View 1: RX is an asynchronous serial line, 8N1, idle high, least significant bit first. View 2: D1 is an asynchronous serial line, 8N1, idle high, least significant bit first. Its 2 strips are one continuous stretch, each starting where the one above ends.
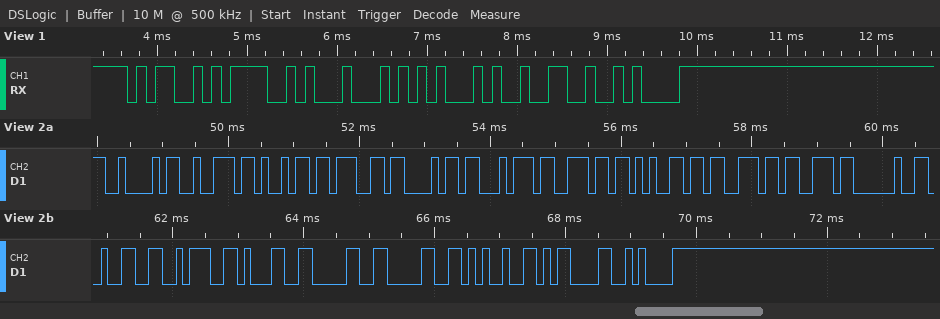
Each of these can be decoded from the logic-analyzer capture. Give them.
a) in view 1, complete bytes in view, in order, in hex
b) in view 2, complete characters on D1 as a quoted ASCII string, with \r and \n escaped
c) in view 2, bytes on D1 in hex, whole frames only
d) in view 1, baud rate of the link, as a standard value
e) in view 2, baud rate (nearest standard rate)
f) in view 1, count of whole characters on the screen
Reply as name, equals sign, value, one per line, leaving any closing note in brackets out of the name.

in view 1, complete bytes in view, in order, in hex = 4D 4F 44 45 32 0A
in view 2, complete characters on D1 as a quoted ASCII string, with \r and \n escaped = "Brightness 2:100%\r\n"
in view 2, bytes on D1 in hex, whole frames only = 0x42 0x72 0x69 0x67 0x68 0x74 0x6E 0x65 0x73 0x73 0x20 0x32 0x3A 0x31 0x30 0x30 0x25 0x0D 0x0A
in view 1, baud rate of the link, as a standard value = 9600 baud
in view 2, baud rate = 9600 baud
in view 1, count of whole characters on the screen = 6
